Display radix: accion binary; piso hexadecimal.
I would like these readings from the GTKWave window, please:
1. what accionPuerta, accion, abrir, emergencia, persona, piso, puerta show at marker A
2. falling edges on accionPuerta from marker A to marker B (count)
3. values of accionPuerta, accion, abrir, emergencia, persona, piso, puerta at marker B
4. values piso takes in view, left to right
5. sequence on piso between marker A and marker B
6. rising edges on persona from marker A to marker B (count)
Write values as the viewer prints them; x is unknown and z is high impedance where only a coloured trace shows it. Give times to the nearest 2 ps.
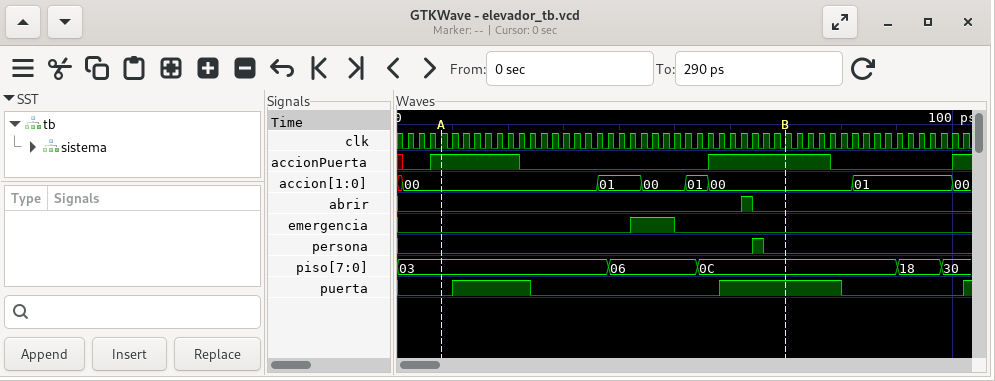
accionPuerta=1, accion=00, abrir=0, emergencia=0, persona=0, piso=03, puerta=0
1
accionPuerta=1, accion=00, abrir=0, emergencia=0, persona=0, piso=0C, puerta=1
03, 06, 0C, 18, 30
03, 06, 0C
1
